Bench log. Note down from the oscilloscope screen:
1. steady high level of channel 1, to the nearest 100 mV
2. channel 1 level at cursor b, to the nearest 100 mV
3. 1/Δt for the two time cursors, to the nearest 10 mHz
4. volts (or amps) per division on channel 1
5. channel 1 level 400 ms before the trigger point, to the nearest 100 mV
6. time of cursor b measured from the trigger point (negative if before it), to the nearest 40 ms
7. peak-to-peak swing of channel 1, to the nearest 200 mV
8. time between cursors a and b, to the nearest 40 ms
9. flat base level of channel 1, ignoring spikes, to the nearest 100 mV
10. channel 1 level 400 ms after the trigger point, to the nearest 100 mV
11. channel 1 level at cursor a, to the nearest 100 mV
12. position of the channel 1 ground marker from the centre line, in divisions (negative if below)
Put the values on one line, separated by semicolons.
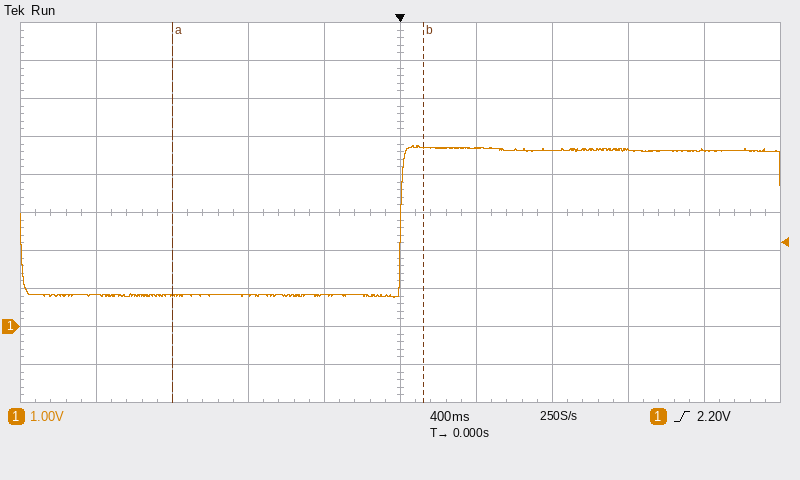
4.6 V; 4.7 V; 760 mHz; 1 V; 800 mV; +120 ms; 4.0 V; 1.32 s; 800 mV; 4.7 V; 800 mV; -3.0 div
